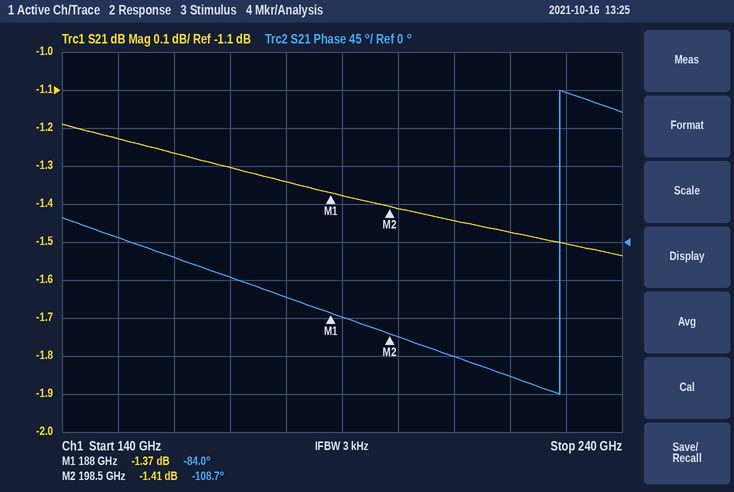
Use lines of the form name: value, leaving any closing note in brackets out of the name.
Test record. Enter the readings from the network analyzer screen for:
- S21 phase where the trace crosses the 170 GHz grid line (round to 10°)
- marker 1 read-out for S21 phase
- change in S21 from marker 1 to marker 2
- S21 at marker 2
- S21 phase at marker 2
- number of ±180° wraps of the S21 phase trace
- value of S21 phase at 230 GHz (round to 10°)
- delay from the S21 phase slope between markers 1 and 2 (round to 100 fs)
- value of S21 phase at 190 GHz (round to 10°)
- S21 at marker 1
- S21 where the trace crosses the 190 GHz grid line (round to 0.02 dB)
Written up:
S21 phase where the trace crosses the 170 GHz grid line: -40°
marker 1 read-out for S21 phase: -84.0°
change in S21 from marker 1 to marker 2: -0.04 dB
S21 at marker 2: -1.41 dB
S21 phase at marker 2: -108.7°
number of ±180° wraps of the S21 phase trace: 1
value of S21 phase at 230 GHz: 180°
delay from the S21 phase slope between markers 1 and 2: 6.5 ps
value of S21 phase at 190 GHz: -90°
S21 at marker 1: -1.37 dB
S21 where the trace crosses the 190 GHz grid line: -1.38 dB
